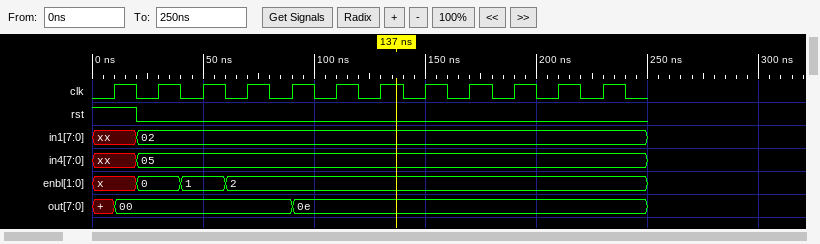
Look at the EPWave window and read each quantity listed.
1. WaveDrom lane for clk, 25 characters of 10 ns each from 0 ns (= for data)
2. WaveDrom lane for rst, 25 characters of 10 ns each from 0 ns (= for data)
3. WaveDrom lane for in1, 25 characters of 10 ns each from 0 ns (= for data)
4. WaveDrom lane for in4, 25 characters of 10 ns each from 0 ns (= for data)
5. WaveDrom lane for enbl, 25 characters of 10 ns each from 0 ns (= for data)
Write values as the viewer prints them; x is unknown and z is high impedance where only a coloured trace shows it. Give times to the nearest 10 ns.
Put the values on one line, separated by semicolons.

{name: 'clk', wave: '0101010101010101010101010'}; {name: 'rst', wave: '1.0......................'}; {name: 'in1', wave: 'x.=......................', data: '02'}; {name: 'in4', wave: 'x.=......................', data: '05'}; {name: 'enbl', wave: 'x.=.=.=..................', data: '0 1 2'}
